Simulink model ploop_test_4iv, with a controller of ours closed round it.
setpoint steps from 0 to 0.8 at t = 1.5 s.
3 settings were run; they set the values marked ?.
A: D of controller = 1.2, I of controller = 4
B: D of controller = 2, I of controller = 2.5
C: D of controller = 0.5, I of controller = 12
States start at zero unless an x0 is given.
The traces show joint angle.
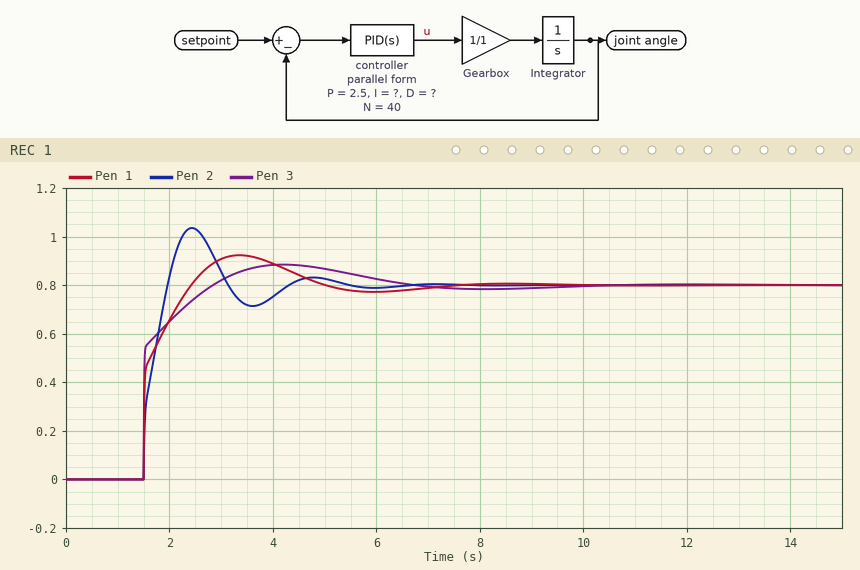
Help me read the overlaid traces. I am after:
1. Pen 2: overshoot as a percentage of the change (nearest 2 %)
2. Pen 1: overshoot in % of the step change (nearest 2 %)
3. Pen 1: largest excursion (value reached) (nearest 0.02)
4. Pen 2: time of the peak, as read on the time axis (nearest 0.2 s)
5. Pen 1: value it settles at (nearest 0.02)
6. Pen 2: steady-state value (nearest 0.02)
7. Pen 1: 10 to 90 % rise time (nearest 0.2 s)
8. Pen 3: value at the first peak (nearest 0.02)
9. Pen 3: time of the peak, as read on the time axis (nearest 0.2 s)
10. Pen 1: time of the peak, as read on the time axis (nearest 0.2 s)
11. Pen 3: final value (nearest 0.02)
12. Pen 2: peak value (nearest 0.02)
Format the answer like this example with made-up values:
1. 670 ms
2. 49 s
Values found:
1. 30 %
2. 16 %
3. 0.92
4. 2.4 s
5. 0.80
6. 0.80
7. 0.6 s
8. 0.88
9. 4.2 s
10. 3.4 s
11. 0.80
12. 1.04
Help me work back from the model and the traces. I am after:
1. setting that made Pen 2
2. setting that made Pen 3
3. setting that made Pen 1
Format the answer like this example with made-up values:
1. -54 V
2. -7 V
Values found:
1. C
2. B
3. A
